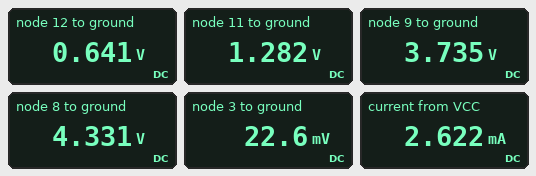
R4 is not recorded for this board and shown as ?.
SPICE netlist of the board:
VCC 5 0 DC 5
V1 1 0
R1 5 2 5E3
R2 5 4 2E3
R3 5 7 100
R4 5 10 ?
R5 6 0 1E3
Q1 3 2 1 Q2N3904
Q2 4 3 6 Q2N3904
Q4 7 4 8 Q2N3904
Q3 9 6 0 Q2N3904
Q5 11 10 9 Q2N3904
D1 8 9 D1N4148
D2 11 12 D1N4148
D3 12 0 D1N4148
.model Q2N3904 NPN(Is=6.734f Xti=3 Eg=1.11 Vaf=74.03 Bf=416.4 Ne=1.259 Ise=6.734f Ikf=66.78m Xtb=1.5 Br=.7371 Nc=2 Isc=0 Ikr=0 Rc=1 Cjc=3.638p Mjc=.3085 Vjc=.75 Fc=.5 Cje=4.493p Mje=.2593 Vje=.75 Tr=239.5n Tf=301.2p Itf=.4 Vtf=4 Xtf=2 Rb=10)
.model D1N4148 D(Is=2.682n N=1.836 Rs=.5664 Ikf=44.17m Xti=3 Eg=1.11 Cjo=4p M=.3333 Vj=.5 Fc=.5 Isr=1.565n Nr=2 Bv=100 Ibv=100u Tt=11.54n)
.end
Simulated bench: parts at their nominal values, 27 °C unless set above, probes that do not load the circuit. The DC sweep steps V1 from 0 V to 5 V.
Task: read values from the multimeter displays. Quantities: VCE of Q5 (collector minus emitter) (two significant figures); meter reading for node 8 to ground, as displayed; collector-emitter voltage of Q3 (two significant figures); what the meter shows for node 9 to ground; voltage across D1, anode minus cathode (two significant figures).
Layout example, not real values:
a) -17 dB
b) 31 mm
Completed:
a) -2.5 V
b) 4.331 V
c) 3.7 V
d) 3.735 V
e) 600 mV
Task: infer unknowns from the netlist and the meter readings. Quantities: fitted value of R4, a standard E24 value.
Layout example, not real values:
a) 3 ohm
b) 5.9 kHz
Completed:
a) 3 kΩ
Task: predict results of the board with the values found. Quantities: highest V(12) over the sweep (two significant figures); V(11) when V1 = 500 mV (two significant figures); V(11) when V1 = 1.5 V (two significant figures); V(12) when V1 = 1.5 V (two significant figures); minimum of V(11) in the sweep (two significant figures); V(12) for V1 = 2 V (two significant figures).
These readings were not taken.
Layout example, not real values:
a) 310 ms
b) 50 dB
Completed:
a) 640 mV
b) 1.3 V
c) 56 mV
d) 28 mV
e) 56 mV
f) 28 mV
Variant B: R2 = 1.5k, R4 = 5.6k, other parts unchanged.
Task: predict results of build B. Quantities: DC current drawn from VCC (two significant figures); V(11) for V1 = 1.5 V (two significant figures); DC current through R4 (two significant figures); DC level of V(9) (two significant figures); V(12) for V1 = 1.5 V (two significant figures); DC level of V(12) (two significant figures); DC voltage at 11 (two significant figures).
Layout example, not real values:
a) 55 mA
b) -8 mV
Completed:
a) 1.8 mA
b) 51 mV
c) 560 µA
d) 3.8 V
e) 25 mV
f) 610 mV
g) 1.2 V
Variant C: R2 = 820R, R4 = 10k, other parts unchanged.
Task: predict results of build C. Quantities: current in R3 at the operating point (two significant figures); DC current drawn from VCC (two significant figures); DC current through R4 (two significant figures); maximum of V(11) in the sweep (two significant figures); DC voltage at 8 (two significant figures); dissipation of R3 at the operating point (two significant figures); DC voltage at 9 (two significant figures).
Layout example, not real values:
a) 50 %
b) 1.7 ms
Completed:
a) 230 µA
b) 1.4 mA
c) 320 µA
d) 1.2 V
e) 4.4 V
f) 5.4 µW
g) 3.8 V
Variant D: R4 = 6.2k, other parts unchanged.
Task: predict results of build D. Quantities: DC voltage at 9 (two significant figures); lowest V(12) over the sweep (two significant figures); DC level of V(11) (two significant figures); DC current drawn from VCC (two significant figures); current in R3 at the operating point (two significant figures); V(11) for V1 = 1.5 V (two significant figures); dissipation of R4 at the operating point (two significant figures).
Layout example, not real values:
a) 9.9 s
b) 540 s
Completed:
a) 3.8 V
b) 25 mV
c) 1.2 V
d) 1.7 mA
e) 370 µA
f) 51 mV
g) 1.6 mW
